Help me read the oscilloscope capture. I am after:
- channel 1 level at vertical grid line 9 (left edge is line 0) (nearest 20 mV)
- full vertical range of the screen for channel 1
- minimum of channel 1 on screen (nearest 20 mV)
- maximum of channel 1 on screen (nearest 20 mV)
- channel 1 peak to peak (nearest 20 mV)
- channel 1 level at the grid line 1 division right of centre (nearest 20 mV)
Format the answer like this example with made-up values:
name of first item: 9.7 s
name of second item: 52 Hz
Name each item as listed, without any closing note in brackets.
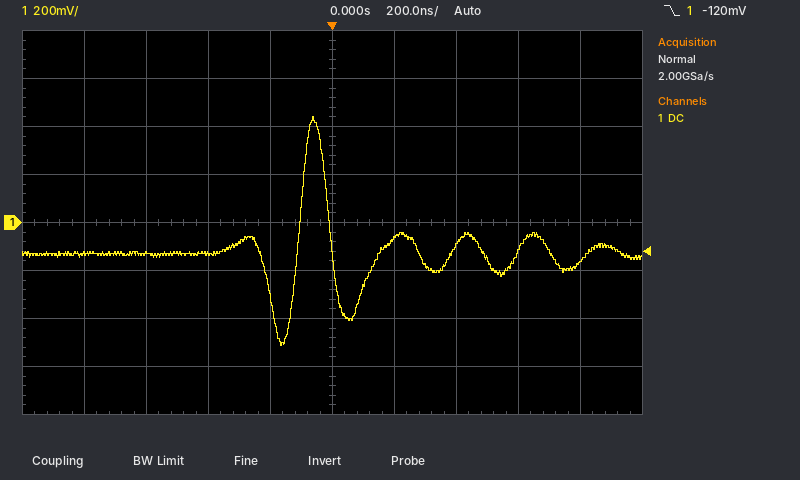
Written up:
channel 1 level at vertical grid line 9 (left edge is line 0): -160 mV
full vertical range of the screen for channel 1: 1.6 V
minimum of channel 1 on screen: -520 mV
maximum of channel 1 on screen: 440 mV
channel 1 peak to peak: 960 mV
channel 1 level at the grid line 1 division right of centre: -60 mV
